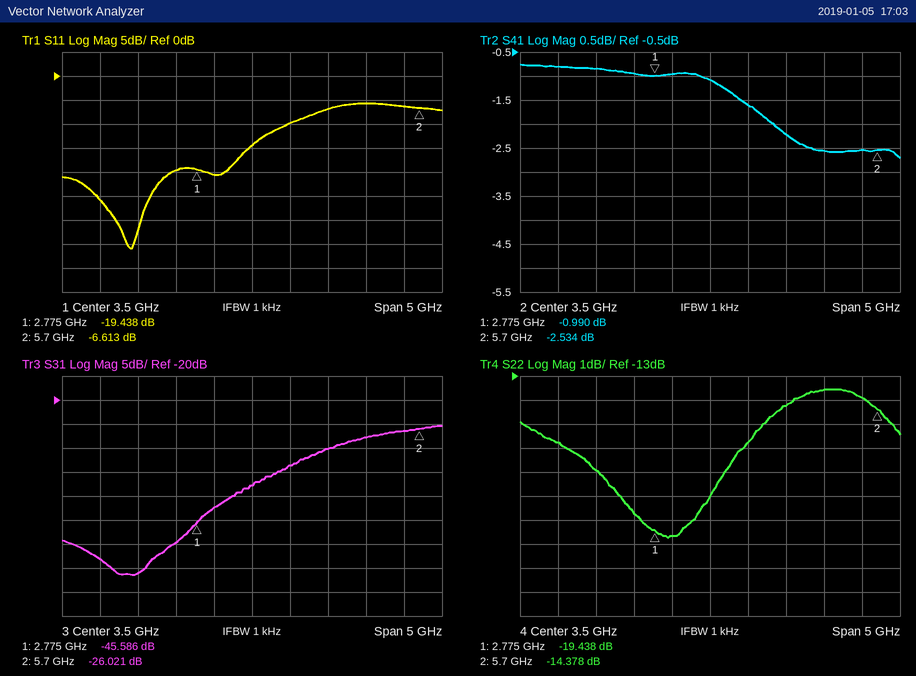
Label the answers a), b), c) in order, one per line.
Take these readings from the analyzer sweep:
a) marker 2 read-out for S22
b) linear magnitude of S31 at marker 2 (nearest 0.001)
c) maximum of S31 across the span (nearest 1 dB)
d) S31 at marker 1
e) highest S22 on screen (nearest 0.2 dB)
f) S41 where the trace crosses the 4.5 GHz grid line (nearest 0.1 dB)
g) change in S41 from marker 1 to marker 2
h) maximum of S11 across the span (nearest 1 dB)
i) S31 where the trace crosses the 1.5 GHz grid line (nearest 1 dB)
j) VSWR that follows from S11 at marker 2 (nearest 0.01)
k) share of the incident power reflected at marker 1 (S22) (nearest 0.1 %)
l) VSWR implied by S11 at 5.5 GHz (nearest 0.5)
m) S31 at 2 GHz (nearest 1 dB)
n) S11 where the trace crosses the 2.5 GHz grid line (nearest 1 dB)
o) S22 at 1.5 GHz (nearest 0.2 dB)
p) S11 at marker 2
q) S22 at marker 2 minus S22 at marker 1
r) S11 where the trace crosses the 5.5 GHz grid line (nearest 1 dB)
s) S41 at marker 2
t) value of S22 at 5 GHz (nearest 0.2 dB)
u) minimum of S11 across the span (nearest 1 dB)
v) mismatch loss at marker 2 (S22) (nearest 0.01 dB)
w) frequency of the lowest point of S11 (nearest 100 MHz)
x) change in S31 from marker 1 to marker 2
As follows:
a) -14.378 dB
b) 0.050
c) -25 dB
d) -45.586 dB
e) -13.6 dB
f) -2.2 dB
g) -1.544 dB
h) -6 dB
i) -53 dB
j) 2.75
k) 1.1 %
l) 3.0
m) -56 dB
n) -20 dB
o) -15.8 dB
p) -6.613 dB
q) 5.060 dB
r) -6 dB
s) -2.534 dB
t) -13.6 dB
u) -36 dB
v) 0.16 dB
w) 1.9 GHz
x) 19.565 dB
